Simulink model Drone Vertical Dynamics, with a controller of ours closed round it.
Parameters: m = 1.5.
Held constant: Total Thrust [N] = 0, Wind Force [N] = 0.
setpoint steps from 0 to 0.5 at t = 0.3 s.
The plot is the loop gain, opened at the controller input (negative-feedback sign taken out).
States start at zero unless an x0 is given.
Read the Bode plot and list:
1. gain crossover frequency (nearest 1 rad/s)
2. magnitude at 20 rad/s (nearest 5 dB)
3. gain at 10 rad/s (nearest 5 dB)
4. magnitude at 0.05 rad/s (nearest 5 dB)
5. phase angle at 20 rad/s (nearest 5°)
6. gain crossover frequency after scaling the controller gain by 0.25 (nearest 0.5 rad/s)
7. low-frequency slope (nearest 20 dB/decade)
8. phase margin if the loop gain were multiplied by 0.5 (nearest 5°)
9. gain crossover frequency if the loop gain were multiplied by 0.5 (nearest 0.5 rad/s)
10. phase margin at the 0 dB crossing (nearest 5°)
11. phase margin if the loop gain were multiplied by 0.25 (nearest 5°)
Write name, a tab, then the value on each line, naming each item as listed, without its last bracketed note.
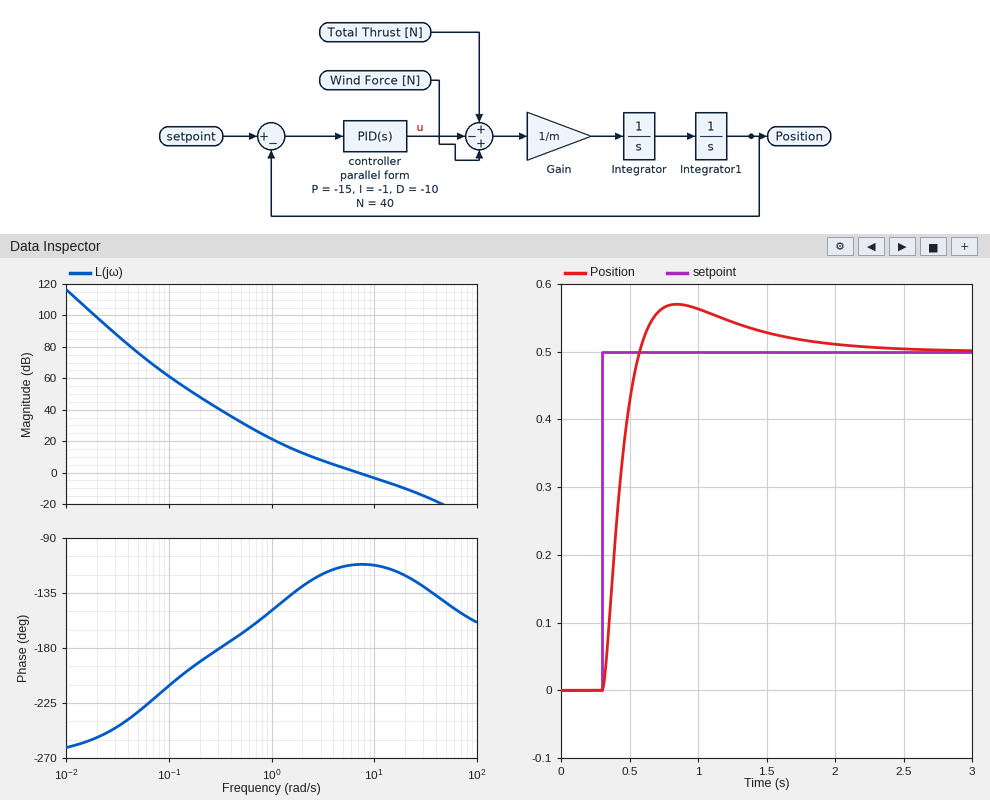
gain crossover frequency	7 rad/s
magnitude at 20 rad/s	-10 dB
gain at 10 rad/s	-5 dB
magnitude at 0.05 rad/s	75 dB
phase angle at 20 rad/s	-120°
gain crossover frequency after scaling the controller gain by 0.25	2.0 rad/s
low-frequency slope	-60 dB/decade
phase margin if the loop gain were multiplied by 0.5	65°
gain crossover frequency if the loop gain were multiplied by 0.5	3.5 rad/s
phase margin at the 0 dB crossing	70°
phase margin if the loop gain were multiplied by 0.25	50°
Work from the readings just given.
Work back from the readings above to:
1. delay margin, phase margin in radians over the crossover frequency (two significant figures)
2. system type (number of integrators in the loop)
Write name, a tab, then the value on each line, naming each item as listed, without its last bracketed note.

delay margin, phase margin in radians over the crossover frequency	0.17 s
system type	3
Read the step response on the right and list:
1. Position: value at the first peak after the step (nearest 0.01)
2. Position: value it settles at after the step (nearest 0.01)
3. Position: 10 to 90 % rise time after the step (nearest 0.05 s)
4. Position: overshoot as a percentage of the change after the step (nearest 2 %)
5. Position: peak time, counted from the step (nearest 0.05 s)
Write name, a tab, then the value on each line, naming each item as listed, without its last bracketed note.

Position: value at the first peak after the step	0.57
Position: value it settles at after the step	0.50
Position: 10 to 90 % rise time after the step	0.20 s
Position: overshoot as a percentage of the change after the step	14 %
Position: peak time, counted from the step	0.55 s
